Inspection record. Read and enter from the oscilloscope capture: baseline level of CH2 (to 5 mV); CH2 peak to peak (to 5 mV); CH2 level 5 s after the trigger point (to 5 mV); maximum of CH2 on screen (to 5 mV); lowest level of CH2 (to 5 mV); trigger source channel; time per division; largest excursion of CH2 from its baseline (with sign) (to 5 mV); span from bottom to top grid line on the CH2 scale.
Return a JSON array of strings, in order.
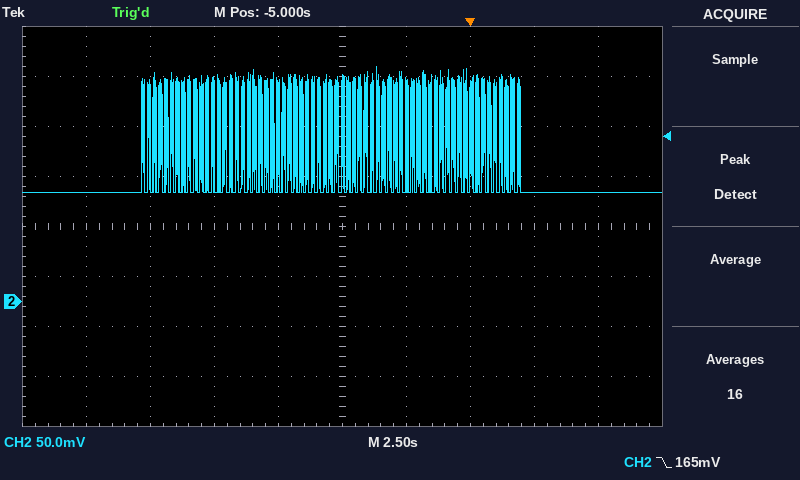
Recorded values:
["110 mV", "125 mV", "110 mV", "235 mV", "110 mV", "CH2", "2.5 s", "+125 mV", "400 mV"]
